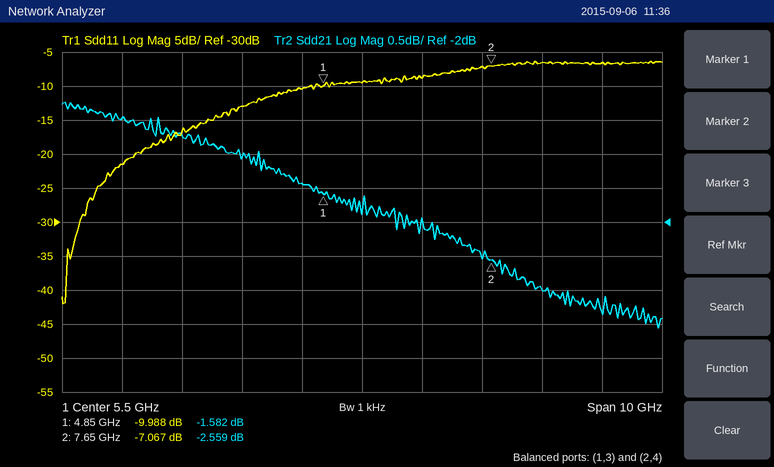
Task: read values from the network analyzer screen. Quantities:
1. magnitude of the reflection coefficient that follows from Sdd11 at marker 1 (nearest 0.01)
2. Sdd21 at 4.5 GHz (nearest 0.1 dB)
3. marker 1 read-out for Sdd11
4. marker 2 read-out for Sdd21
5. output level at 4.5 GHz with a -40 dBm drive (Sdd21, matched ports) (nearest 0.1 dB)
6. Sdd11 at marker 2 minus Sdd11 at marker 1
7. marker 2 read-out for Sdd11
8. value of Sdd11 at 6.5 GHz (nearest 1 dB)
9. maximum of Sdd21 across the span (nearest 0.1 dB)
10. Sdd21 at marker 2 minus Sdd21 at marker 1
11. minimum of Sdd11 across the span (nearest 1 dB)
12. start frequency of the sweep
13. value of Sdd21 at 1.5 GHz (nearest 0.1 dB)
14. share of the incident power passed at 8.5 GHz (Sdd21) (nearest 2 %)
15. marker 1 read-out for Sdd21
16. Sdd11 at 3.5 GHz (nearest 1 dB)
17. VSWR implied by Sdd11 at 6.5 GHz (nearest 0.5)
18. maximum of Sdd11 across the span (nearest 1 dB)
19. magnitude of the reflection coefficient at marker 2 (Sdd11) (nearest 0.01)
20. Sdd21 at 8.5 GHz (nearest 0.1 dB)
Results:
0.32
-1.4 dB
-9.988 dB
-2.559 dB
-41.4 dBm
2.921 dB
-7.067 dB
-9 dB
-0.2 dB
-0.977 dB
-42 dB
500 MHz
-0.5 dB
50 %
-1.582 dB
-13 dB
2.0
-6 dB
0.44
-3.0 dB
